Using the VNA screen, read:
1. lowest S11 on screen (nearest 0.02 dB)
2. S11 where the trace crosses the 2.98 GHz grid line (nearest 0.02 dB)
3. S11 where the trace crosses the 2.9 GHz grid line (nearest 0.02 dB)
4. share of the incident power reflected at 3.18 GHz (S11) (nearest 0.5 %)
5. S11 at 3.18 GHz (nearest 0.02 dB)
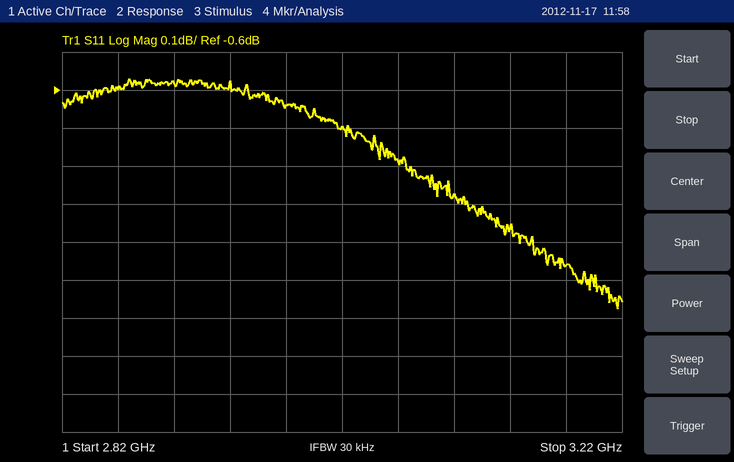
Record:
-1.18 dB
-0.64 dB
-0.58 dB
78.5 %
-1.06 dB
